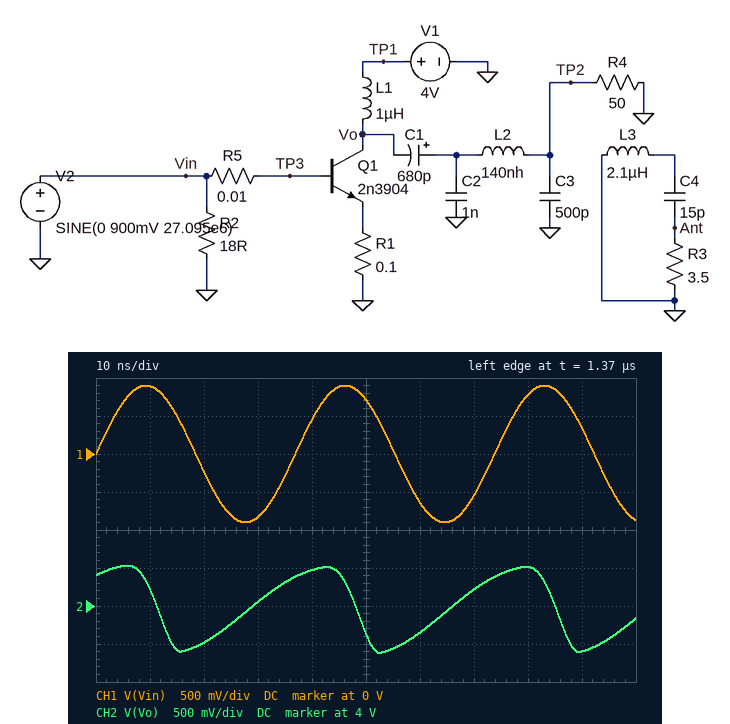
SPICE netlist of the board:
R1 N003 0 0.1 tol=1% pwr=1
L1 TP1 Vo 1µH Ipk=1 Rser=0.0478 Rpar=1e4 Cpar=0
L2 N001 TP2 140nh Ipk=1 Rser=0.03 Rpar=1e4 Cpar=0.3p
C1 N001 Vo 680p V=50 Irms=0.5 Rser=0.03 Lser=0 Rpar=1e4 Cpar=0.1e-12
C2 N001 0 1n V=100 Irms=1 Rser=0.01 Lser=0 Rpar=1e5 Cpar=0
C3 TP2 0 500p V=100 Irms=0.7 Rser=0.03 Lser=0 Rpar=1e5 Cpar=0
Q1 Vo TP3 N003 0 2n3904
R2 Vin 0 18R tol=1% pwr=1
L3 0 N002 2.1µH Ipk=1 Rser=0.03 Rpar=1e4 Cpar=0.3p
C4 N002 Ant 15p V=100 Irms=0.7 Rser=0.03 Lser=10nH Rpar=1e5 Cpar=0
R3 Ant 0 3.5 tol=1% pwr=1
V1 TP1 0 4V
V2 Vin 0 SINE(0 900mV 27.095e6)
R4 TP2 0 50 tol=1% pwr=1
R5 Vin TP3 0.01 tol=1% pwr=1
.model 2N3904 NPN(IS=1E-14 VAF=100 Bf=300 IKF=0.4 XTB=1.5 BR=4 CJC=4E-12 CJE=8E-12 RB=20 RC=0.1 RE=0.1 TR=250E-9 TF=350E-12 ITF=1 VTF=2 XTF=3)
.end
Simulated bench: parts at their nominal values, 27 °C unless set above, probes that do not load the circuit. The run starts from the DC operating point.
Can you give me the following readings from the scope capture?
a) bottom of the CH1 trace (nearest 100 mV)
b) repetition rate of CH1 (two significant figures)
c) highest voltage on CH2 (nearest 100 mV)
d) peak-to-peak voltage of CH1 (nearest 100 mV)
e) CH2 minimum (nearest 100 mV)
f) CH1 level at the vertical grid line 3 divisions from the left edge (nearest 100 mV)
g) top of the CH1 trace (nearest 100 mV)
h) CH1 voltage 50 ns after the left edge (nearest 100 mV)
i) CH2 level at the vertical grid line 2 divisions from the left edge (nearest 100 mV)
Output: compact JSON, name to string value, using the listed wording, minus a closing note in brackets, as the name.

{"bottom of the CH1 trace": "-900 mV", "repetition rate of CH1": "27 MHz", "highest voltage on CH2": "4.5 V", "peak-to-peak voltage of CH1": "1.8 V", "CH2 minimum": "3.4 V", "CH1 level at the vertical grid line 3 divisions from the left edge": "-800 mV", "top of the CH1 trace": "900 mV", "CH1 voltage 50 ns after the left edge": "700 mV", "CH2 level at the vertical grid line 2 divisions from the left edge": "3.5 V"}
